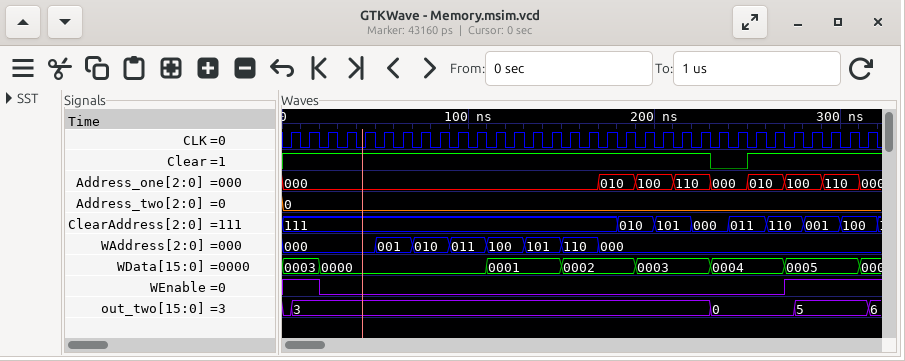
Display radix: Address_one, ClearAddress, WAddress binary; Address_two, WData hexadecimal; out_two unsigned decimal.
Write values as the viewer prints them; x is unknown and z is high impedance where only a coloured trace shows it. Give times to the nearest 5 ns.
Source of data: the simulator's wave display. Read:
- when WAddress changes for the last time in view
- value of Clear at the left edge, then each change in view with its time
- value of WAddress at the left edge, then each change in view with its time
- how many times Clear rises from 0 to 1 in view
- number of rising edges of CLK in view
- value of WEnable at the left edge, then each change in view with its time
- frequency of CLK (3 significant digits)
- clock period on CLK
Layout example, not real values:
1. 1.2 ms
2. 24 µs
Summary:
1. 170 ns
2. 1, 0 at 230 ns, 1 at 250 ns
3. 000, 001 at 50 ns, 010 at 70 ns, 011 at 90 ns, 100 at 110 ns, 101 at 130 ns, 110 at 150 ns, 000 at 170 ns
4. 1
5. 32
6. 1, 0 at 20 ns, 1 at 270 ns
7. 100 MHz
8. 10 ns
